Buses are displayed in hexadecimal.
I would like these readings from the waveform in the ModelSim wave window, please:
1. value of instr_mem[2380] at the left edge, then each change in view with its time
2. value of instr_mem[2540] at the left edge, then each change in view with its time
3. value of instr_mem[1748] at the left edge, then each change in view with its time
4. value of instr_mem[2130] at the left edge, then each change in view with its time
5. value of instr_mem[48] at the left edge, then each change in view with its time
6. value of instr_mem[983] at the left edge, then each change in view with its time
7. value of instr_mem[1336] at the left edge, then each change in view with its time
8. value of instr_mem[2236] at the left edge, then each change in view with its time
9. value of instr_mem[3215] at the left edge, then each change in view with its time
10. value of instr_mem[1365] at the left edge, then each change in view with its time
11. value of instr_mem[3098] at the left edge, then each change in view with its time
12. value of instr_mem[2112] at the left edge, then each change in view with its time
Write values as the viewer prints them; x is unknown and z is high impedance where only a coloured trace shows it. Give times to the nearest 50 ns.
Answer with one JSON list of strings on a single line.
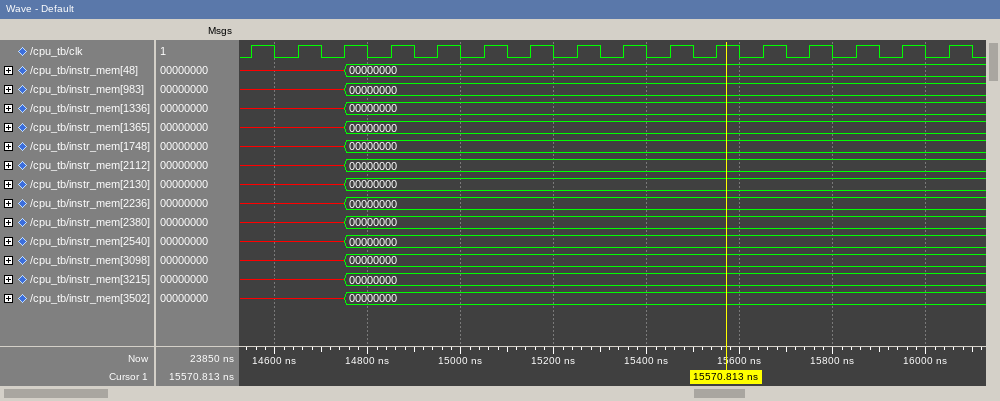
["x, 00000000 at 14750 ns", "x, 00000000 at 14750 ns", "x, 00000000 at 14750 ns", "x, 00000000 at 14750 ns", "x, 00000000 at 14750 ns", "x, 00000000 at 14750 ns", "x, 00000000 at 14750 ns", "x, 00000000 at 14750 ns", "x, 00000000 at 14750 ns", "x, 00000000 at 14750 ns", "x, 00000000 at 14750 ns", "x, 00000000 at 14750 ns"]
